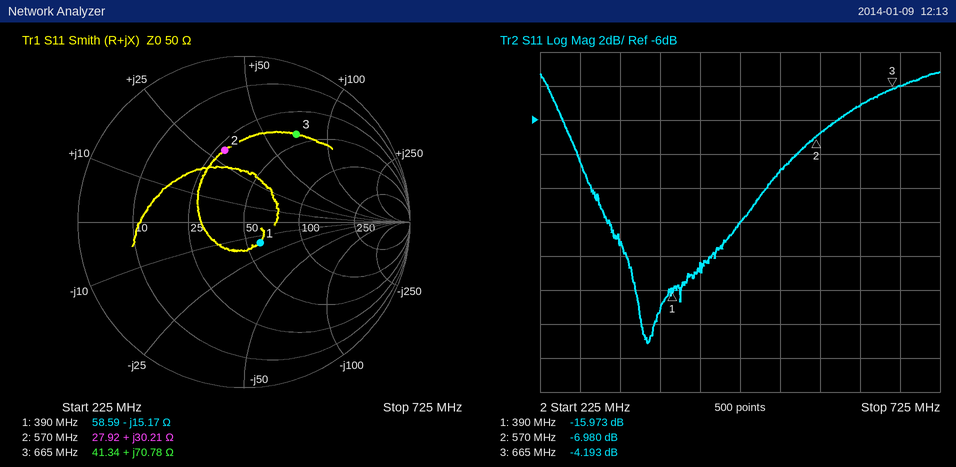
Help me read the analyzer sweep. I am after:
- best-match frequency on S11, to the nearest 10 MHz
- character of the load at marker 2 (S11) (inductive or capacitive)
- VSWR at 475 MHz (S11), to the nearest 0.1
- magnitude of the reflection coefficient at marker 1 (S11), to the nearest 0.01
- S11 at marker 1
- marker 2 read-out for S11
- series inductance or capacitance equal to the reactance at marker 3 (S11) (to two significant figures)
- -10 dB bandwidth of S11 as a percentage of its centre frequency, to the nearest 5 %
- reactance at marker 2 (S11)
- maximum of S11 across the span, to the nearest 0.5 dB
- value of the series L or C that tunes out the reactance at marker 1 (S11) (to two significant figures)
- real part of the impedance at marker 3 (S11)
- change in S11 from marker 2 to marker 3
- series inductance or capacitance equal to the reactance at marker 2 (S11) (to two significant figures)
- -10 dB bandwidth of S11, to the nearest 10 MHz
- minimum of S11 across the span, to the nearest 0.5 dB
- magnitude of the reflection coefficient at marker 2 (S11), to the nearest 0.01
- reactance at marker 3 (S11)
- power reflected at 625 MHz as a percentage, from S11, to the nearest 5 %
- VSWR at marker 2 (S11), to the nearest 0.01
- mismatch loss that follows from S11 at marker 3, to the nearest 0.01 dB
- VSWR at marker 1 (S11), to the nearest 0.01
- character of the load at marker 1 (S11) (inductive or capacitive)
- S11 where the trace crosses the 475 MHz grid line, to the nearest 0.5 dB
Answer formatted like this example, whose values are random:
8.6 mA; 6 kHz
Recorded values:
360 MHz; inductive; 1.7; 0.16; -15.973 dB; -6.980 dB; 17 nH; 55 %; +30.21 Ω; -3.0 dB; 6.2 nH; 41.34 Ω; 2.787 dB; 8.4 nH; 220 MHz; -19.0 dB; 0.45; +70.78 Ω; 30 %; 2.62; 2.08 dB; 1.38; capacitive; -12.0 dB
